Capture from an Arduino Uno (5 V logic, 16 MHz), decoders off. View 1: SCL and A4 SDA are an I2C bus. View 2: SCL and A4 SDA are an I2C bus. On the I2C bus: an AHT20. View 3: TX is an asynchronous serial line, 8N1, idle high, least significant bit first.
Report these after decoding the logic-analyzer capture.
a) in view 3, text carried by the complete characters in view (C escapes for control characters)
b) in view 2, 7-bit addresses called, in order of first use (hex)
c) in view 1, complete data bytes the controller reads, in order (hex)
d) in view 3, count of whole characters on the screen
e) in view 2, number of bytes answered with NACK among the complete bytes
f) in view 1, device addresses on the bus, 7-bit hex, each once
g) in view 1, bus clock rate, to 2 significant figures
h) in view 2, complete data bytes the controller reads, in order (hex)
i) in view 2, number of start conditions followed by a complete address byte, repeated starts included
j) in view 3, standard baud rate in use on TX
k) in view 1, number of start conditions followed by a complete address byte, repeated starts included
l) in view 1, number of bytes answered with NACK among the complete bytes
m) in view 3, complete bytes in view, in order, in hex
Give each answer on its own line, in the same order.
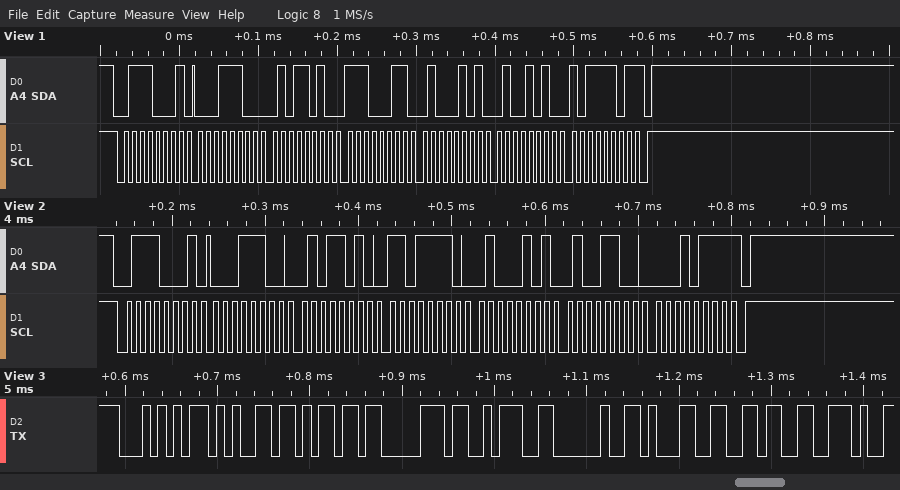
"Temp: 16."
0x38
1C 5A E3 45 4A BD
9
1
0x38
100 kHz
1C 5A DE 45 4C 17
1
115200 baud
1
1
54 65 6D 70 3A 20 31 36 2E
